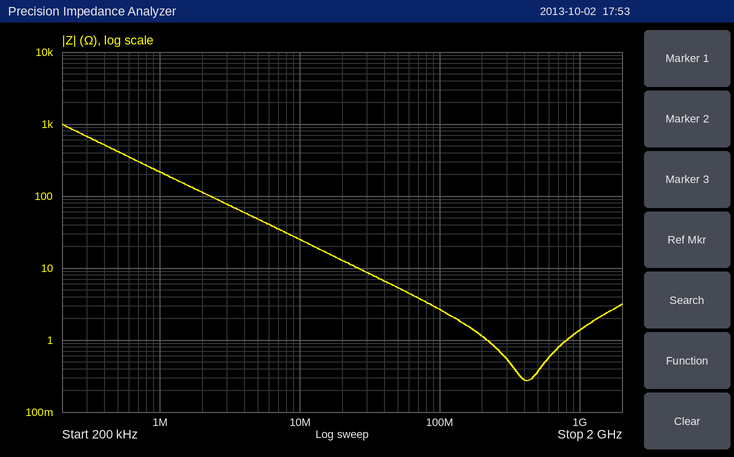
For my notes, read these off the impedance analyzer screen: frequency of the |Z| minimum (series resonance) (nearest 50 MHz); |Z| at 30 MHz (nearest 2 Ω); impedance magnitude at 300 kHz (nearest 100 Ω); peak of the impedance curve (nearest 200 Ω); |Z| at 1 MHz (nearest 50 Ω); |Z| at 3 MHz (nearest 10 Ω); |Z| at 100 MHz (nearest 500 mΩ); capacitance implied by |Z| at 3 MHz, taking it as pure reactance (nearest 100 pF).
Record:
400 MHz
8 Ω
700 Ω
1.0 kΩ
200 Ω
80 Ω
2.5 Ω
700 pF
